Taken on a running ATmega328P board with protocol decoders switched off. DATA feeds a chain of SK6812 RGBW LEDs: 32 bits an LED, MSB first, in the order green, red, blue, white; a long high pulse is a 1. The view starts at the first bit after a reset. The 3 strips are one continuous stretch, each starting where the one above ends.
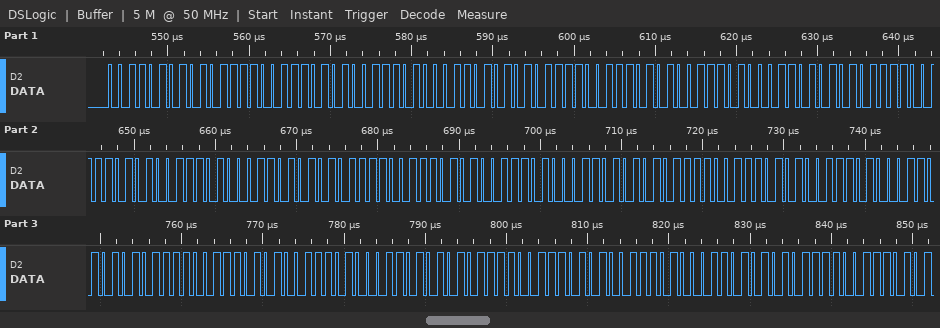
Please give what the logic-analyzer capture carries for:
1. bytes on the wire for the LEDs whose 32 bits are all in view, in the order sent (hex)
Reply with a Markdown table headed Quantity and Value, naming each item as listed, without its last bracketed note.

| Quantity | Value |
|---|---|
| bytes on the wire for the LEDs whose 32 bits are all in view, in the order sent | 35 5E 75 3A 35 5E 75 3A 35 5E 75 3A 35 5E 75 3A 35 5E 75 3A 35 5E 75 3A 35 5E 75 3A |
